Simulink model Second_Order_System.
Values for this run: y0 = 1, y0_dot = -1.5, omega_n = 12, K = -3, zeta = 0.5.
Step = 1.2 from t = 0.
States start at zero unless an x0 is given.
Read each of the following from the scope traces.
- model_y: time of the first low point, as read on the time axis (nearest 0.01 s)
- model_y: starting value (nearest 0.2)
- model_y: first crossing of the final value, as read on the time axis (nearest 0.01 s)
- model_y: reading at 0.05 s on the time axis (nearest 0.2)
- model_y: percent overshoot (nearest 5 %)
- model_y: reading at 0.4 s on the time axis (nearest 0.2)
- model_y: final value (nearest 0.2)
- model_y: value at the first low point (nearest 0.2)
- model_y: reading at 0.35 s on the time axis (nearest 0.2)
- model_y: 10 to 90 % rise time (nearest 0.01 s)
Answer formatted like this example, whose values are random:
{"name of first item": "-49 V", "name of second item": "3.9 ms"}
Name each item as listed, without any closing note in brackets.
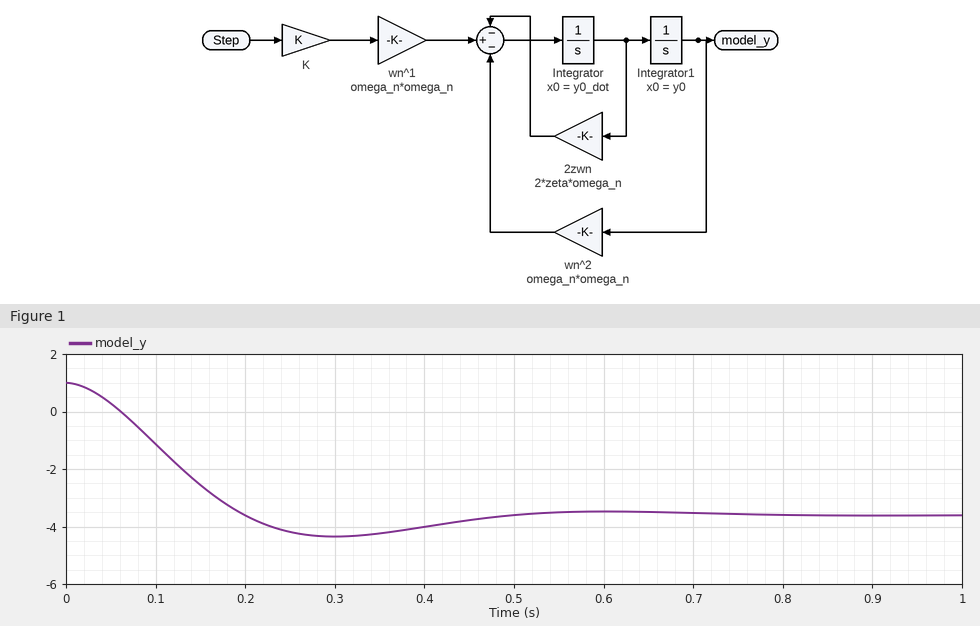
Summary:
{"model_y: time of the first low point, as read on the time axis": "0.30 s", "model_y: starting value": "1.0", "model_y: first crossing of the final value, as read on the time axis": "0.20 s", "model_y: reading at 0.05 s on the time axis": "0.2", "model_y: percent overshoot": "15 %", "model_y: reading at 0.4 s on the time axis": "-4.0", "model_y: final value": "-3.6", "model_y: value at the first low point": "-4.4", "model_y: reading at 0.35 s on the time axis": "-4.2", "model_y: 10 to 90 % rise time": "0.14 s"}
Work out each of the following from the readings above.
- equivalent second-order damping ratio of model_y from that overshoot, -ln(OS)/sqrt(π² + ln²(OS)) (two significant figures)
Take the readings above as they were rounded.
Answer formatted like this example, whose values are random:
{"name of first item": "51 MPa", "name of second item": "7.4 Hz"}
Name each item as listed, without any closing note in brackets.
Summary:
{"equivalent second-order damping ratio of model_y from that overshoot, -ln(OS)/sqrt(π² + ln²(OS))": "0.52"}
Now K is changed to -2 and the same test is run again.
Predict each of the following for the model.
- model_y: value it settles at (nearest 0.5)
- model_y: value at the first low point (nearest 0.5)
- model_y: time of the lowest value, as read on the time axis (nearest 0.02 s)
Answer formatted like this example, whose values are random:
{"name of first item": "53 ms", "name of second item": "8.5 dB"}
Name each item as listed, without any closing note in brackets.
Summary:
{"model_y: value it settles at": "-2.5", "model_y: value at the first low point": "-3.0", "model_y: time of the lowest value, as read on the time axis": "0.30 s"}
